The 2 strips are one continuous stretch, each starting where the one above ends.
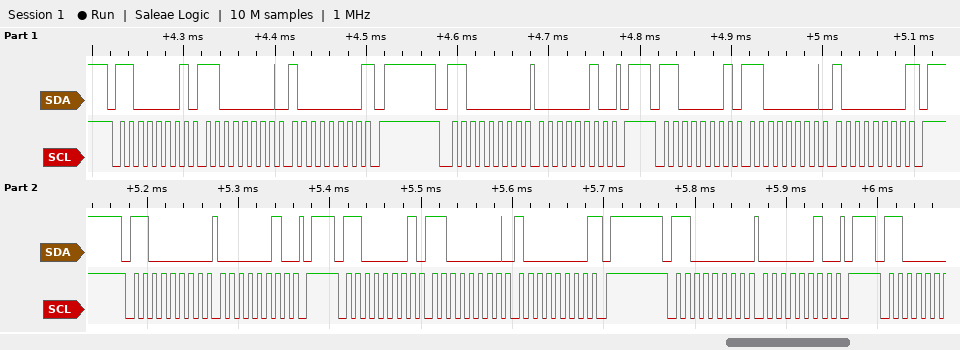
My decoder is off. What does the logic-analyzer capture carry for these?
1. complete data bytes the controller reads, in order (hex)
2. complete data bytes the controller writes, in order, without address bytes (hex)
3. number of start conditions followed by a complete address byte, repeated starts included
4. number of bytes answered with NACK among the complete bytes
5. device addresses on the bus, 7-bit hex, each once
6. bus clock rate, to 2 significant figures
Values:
C0 80 C0 80 C0 80
02 02 02
6
3
0x60
100 kHz
